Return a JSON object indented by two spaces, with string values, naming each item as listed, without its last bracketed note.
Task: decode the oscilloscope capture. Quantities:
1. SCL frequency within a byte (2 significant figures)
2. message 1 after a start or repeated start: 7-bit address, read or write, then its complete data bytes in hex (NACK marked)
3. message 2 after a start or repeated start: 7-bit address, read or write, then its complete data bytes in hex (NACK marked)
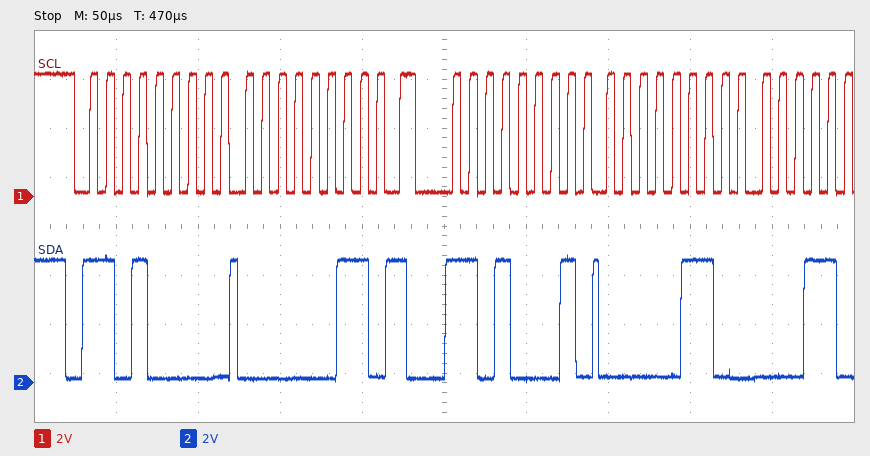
{
  "SCL frequency within a byte": "100 kHz",
  "message 1 after a start or repeated start: 7-bit address, read or write, then its complete data bytes in hex": "0x68 write: 03",
  "message 2 after a start or repeated start: 7-bit address, read or write, then its complete data bytes in hex": "0x68 read: 06"
}
